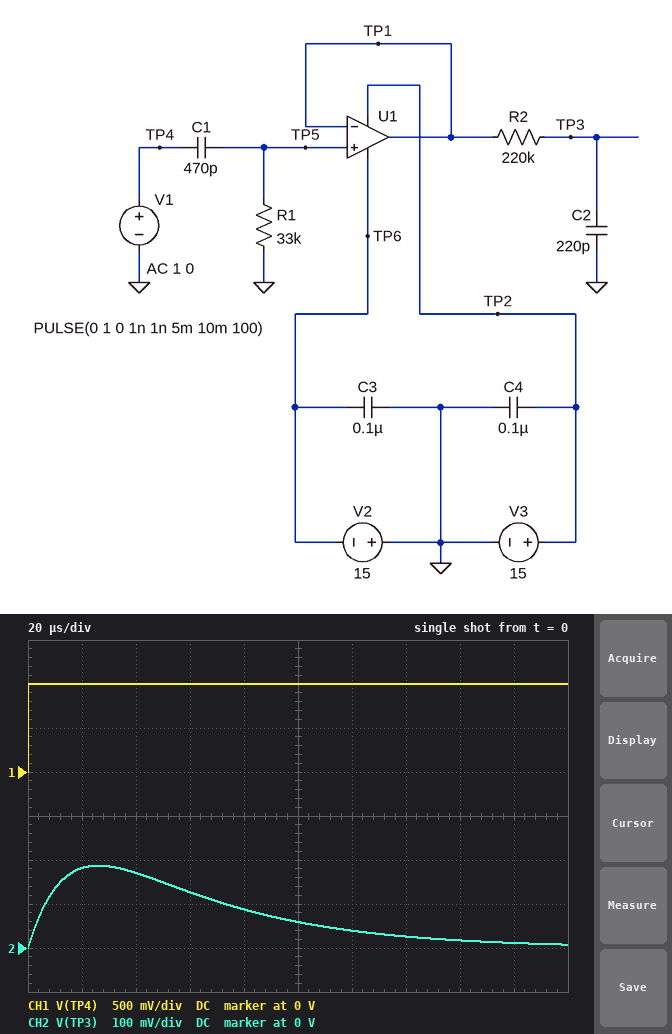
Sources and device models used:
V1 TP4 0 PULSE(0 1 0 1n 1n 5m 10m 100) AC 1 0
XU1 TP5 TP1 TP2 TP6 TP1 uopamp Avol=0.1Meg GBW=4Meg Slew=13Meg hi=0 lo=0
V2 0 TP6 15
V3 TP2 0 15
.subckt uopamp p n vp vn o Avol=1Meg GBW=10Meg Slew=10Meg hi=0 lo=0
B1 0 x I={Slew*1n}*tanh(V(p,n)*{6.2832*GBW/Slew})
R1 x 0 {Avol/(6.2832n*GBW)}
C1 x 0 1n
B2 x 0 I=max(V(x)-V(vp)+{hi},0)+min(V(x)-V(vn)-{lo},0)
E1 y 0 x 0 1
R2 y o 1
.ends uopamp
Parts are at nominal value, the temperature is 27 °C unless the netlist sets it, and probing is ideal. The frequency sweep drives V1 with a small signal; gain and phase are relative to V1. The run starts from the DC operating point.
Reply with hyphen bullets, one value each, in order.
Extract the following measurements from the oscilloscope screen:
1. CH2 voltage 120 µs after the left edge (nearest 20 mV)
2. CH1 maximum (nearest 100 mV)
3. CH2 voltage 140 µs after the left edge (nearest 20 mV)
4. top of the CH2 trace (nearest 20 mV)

- 40 mV
- 1.0 V
- 20 mV
- 180 mV
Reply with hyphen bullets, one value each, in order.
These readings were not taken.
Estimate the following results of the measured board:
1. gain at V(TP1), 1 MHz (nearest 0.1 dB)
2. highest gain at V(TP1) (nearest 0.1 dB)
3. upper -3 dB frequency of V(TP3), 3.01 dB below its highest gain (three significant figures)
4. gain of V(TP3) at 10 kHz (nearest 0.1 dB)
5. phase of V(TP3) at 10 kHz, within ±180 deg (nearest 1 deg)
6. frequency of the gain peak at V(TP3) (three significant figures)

- -0.3 dB
- 0 dB
- 15.7 kHz
- -13.2 dB
- -26 deg
- 5.81 kHz
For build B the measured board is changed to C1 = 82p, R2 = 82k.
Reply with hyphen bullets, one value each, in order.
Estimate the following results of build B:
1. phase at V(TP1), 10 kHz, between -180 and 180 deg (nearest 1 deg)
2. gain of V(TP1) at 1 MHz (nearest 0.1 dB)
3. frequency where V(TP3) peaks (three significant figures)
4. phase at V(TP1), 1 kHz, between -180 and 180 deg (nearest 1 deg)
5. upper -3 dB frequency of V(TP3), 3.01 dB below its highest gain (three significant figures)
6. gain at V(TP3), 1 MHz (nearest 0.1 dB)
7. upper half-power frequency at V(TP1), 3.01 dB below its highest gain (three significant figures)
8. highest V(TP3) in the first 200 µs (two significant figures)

- 80 deg
- -0.3 dB
- 22.8 kHz
- 89 deg
- 74.6 kHz
- -41.4 dB
- 4.12 MHz
- 110 mV
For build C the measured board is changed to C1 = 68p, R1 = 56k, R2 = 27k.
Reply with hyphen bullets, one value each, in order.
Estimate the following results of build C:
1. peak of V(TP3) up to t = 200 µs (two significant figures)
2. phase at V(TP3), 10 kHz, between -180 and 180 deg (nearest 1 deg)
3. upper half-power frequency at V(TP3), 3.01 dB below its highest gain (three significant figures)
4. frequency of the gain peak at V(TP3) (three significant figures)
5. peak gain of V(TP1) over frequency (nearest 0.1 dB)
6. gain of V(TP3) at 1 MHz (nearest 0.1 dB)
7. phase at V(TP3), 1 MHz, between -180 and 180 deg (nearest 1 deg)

- 290 mV
- 56 deg
- 82.2 kHz
- 33.5 kHz
- -0.1 dB
- -31.7 dB
- -100 deg
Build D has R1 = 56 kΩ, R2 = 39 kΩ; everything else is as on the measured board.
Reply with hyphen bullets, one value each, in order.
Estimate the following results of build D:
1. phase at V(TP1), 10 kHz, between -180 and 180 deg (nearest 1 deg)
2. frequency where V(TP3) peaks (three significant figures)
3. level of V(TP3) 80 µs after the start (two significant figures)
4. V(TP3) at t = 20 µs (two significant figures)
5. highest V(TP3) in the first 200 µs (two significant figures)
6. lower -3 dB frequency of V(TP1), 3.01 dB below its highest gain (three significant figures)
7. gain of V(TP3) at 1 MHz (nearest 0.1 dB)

- 31 deg
- 10.6 kHz
- 71 mV
- 550 mV
- 580 mV
- 6.03 kHz
- -34.9 dB
